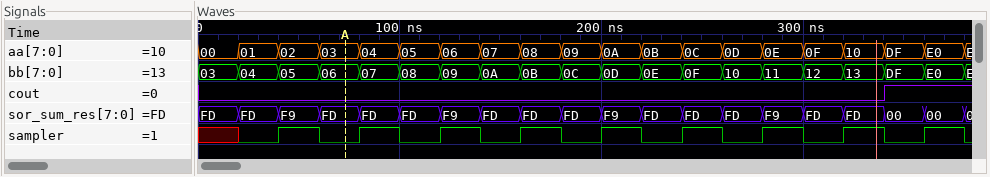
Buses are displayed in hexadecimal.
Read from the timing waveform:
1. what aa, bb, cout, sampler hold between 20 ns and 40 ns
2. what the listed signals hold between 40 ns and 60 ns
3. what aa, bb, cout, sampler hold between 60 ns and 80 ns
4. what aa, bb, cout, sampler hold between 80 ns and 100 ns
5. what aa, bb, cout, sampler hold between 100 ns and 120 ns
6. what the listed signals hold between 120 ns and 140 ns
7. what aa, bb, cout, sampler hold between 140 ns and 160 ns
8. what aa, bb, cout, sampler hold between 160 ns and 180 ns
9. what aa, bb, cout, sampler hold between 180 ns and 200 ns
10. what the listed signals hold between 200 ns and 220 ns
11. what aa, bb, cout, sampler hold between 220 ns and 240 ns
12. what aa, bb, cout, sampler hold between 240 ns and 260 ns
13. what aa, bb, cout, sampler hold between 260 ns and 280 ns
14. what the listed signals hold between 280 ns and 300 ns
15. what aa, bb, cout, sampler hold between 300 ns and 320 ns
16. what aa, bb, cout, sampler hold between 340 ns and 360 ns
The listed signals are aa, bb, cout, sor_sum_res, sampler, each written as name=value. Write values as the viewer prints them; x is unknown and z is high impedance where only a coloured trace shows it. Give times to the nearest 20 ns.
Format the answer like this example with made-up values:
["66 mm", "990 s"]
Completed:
["aa=01, bb=04, cout=0, sampler=0", "aa=02, bb=05, cout=0, sor_sum_res=F9, sampler=1", "aa=03, bb=06, cout=0, sampler=0", "aa=04, bb=07, cout=0, sampler=1", "aa=05, bb=08, cout=0, sampler=0", "aa=06, bb=09, cout=0, sor_sum_res=F9, sampler=1", "aa=07, bb=0A, cout=0, sampler=0", "aa=08, bb=0B, cout=0, sampler=1", "aa=09, bb=0C, cout=0, sampler=0", "aa=0A, bb=0D, cout=0, sor_sum_res=F9, sampler=1", "aa=0B, bb=0E, cout=0, sampler=0", "aa=0C, bb=0F, cout=0, sampler=1", "aa=0D, bb=10, cout=0, sampler=0", "aa=0E, bb=11, cout=0, sor_sum_res=F9, sampler=1", "aa=0F, bb=12, cout=0, sampler=0", "aa=DF, bb=DF, cout=1, sampler=0"]
